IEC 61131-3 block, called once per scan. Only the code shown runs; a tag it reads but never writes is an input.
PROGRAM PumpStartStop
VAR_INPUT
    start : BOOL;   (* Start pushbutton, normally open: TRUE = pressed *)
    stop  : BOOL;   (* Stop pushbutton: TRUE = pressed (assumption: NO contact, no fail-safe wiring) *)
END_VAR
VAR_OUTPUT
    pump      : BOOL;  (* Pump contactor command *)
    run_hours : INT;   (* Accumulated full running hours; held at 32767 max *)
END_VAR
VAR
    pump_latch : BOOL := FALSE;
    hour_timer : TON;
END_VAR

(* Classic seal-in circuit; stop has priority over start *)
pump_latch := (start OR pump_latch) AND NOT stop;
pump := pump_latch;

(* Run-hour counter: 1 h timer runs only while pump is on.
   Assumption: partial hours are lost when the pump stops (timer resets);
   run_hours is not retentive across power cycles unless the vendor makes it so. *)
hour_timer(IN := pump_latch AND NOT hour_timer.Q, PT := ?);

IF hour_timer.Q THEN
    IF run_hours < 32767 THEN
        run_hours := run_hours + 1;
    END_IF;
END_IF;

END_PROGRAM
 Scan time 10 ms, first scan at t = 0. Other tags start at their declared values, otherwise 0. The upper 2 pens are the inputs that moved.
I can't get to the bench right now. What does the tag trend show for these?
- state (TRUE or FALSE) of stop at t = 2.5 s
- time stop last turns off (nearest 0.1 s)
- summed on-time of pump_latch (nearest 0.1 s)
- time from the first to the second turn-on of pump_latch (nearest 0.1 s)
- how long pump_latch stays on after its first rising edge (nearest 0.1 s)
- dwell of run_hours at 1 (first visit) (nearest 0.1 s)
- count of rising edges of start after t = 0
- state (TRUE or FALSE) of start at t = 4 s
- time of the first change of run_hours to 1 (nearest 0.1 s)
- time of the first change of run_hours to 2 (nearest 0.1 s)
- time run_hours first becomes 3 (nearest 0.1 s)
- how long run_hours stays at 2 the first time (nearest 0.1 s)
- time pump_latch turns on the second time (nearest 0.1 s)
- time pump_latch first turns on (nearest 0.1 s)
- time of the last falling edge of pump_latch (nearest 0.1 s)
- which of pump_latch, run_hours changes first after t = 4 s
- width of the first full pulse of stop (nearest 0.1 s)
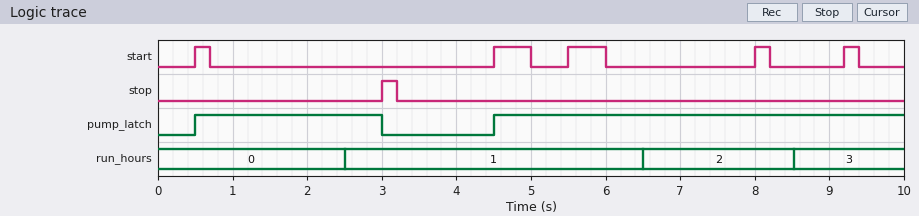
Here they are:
FALSE
3.2 s
8.0 s
4.0 s
2.5 s
4.0 s
5
FALSE
2.5 s
6.5 s
8.5 s
2.0 s
4.5 s
0.5 s
3.0 s
pump_latch
0.2 s
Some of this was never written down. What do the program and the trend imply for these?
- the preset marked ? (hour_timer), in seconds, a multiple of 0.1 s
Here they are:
2.0 s
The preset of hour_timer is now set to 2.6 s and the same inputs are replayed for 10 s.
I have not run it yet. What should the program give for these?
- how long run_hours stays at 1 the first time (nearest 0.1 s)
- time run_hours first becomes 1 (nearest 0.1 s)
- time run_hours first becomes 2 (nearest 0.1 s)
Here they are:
2.6 s
7.1 s
9.7 s
